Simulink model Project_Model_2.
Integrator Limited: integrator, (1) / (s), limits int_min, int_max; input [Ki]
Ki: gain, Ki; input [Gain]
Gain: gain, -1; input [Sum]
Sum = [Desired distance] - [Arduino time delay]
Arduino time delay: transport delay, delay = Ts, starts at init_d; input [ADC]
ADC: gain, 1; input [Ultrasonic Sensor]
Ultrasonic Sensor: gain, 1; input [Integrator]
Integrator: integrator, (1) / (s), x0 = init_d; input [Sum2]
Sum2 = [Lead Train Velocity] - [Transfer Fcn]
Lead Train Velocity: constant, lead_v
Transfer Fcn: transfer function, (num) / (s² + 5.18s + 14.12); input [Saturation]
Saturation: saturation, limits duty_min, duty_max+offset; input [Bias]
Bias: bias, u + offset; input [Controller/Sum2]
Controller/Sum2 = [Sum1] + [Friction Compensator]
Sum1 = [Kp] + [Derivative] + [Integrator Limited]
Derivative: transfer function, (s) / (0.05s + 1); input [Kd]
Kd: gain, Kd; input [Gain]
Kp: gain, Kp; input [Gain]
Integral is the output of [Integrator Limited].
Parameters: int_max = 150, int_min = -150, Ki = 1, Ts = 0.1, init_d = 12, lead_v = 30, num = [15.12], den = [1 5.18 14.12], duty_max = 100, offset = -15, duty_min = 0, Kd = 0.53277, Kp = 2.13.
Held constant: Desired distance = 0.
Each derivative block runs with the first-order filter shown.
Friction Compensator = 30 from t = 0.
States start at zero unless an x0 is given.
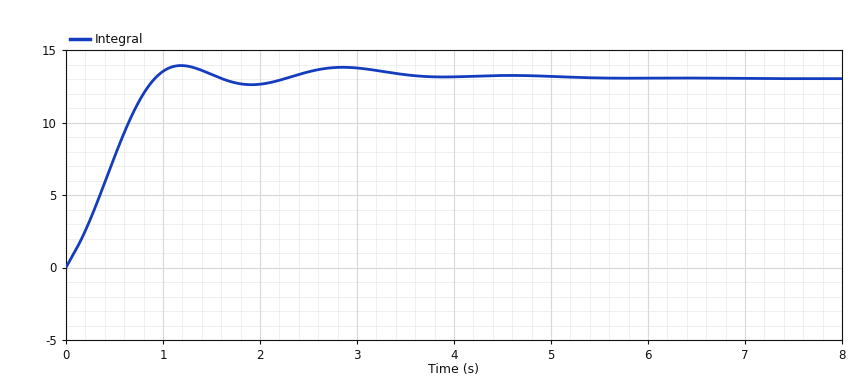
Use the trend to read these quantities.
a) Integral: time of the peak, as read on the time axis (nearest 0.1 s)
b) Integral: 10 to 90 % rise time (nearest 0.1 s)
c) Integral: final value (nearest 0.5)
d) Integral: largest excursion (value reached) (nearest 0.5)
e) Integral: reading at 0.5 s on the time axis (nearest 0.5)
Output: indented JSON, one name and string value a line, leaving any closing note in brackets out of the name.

{
  "Integral: time of the peak, as read on the time axis": "1.2 s",
  "Integral: 10 to 90 % rise time": "0.7 s",
  "Integral: final value": "13.0",
  "Integral: largest excursion (value reached)": "14.0",
  "Integral: reading at 0.5 s on the time axis": "7.5"
}
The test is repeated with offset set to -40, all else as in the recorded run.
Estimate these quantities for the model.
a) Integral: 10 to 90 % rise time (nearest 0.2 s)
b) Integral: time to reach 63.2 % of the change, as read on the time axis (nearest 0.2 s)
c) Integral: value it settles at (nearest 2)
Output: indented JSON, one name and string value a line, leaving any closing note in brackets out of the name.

{
  "Integral: 10 to 90 % rise time": "3.0 s",
  "Integral: time to reach 63.2 % of the change, as read on the time axis": "1.6 s",
  "Integral: value it settles at": "38"
}
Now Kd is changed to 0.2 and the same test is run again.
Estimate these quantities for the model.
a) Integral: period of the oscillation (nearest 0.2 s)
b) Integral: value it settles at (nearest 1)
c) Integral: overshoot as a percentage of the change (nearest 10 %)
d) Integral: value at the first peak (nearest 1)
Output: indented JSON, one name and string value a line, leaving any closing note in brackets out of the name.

{
  "Integral: period of the oscillation": "2.4 s",
  "Integral: value it settles at": "13",
  "Integral: overshoot as a percentage of the change": "20 %",
  "Integral: value at the first peak": "16"
}
